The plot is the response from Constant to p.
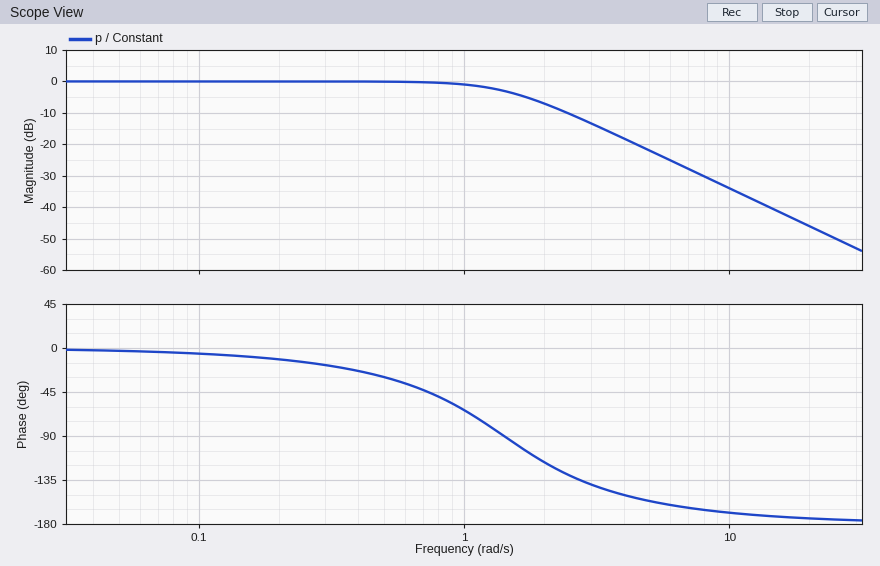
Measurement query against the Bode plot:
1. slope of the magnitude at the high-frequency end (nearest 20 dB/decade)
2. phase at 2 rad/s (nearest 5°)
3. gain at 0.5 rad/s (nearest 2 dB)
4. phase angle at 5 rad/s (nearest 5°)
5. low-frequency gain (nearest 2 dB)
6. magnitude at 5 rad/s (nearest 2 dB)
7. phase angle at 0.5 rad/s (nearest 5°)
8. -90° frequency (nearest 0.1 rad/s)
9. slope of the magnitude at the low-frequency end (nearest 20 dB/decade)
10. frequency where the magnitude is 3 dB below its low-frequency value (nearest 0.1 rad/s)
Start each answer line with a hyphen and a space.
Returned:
- -40 dB/decade
- -115°
- 0 dB
- -155°
- 0 dB
- -22 dB
- -30°
- 1.4 rad/s
- 0 dB/decade
- 1.4 rad/s
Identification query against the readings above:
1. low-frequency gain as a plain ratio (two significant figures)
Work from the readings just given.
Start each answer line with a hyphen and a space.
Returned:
- 1.0
